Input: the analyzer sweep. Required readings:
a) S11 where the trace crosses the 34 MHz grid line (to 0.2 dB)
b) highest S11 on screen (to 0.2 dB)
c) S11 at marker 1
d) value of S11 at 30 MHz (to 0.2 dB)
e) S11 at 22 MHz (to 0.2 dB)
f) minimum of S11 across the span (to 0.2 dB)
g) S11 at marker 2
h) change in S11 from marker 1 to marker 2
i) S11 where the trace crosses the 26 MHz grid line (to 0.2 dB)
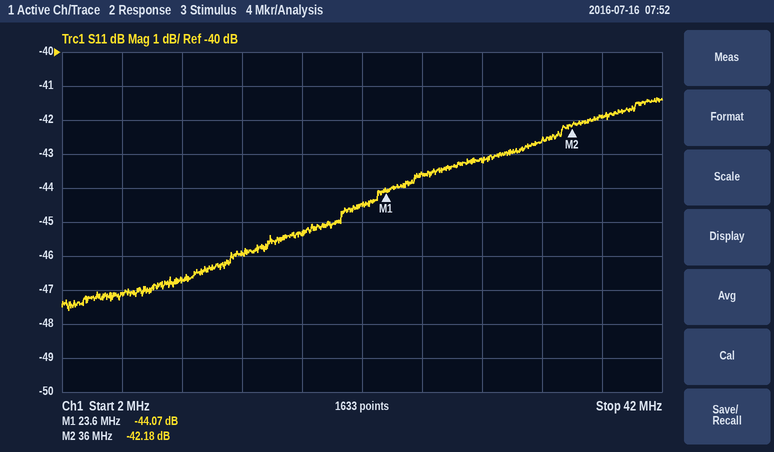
-42.6 dB
-41.4 dB
-44.07 dB
-43.2 dB
-44.4 dB
-47.6 dB
-42.18 dB
1.89 dB
-43.6 dB
